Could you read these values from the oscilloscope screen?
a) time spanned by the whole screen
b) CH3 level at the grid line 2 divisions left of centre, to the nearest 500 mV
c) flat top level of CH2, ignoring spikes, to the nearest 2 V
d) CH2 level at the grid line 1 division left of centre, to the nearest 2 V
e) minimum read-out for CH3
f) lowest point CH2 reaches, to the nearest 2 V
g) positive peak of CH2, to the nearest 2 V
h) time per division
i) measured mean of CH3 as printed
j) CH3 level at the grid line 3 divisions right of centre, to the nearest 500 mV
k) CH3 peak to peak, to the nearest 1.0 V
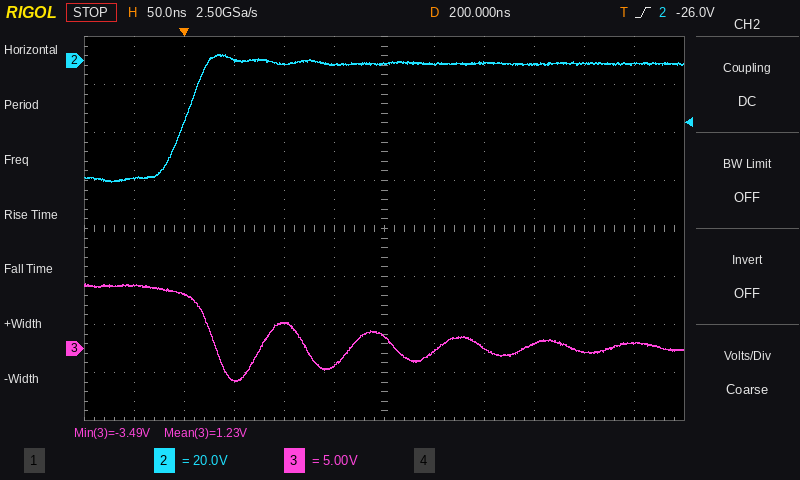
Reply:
600 ns
2.5 V
-2 V
-2 V
-3.49 V
-50 V
2 V
50 ns
1.23 V
500 mV
10.0 V
